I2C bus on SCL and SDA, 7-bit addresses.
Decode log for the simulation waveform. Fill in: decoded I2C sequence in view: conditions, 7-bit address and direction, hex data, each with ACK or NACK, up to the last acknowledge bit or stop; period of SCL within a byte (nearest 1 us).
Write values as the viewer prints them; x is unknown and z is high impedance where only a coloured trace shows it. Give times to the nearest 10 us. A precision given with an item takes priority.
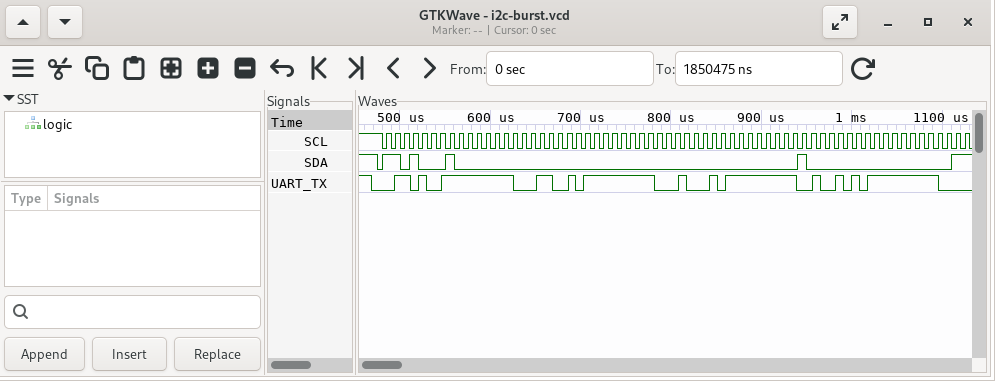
start, address 68 read ACK, 00 ACK, 00 ACK, 00 ACK, 00 ACK, 40 ACK, 00 ACK
10 us
